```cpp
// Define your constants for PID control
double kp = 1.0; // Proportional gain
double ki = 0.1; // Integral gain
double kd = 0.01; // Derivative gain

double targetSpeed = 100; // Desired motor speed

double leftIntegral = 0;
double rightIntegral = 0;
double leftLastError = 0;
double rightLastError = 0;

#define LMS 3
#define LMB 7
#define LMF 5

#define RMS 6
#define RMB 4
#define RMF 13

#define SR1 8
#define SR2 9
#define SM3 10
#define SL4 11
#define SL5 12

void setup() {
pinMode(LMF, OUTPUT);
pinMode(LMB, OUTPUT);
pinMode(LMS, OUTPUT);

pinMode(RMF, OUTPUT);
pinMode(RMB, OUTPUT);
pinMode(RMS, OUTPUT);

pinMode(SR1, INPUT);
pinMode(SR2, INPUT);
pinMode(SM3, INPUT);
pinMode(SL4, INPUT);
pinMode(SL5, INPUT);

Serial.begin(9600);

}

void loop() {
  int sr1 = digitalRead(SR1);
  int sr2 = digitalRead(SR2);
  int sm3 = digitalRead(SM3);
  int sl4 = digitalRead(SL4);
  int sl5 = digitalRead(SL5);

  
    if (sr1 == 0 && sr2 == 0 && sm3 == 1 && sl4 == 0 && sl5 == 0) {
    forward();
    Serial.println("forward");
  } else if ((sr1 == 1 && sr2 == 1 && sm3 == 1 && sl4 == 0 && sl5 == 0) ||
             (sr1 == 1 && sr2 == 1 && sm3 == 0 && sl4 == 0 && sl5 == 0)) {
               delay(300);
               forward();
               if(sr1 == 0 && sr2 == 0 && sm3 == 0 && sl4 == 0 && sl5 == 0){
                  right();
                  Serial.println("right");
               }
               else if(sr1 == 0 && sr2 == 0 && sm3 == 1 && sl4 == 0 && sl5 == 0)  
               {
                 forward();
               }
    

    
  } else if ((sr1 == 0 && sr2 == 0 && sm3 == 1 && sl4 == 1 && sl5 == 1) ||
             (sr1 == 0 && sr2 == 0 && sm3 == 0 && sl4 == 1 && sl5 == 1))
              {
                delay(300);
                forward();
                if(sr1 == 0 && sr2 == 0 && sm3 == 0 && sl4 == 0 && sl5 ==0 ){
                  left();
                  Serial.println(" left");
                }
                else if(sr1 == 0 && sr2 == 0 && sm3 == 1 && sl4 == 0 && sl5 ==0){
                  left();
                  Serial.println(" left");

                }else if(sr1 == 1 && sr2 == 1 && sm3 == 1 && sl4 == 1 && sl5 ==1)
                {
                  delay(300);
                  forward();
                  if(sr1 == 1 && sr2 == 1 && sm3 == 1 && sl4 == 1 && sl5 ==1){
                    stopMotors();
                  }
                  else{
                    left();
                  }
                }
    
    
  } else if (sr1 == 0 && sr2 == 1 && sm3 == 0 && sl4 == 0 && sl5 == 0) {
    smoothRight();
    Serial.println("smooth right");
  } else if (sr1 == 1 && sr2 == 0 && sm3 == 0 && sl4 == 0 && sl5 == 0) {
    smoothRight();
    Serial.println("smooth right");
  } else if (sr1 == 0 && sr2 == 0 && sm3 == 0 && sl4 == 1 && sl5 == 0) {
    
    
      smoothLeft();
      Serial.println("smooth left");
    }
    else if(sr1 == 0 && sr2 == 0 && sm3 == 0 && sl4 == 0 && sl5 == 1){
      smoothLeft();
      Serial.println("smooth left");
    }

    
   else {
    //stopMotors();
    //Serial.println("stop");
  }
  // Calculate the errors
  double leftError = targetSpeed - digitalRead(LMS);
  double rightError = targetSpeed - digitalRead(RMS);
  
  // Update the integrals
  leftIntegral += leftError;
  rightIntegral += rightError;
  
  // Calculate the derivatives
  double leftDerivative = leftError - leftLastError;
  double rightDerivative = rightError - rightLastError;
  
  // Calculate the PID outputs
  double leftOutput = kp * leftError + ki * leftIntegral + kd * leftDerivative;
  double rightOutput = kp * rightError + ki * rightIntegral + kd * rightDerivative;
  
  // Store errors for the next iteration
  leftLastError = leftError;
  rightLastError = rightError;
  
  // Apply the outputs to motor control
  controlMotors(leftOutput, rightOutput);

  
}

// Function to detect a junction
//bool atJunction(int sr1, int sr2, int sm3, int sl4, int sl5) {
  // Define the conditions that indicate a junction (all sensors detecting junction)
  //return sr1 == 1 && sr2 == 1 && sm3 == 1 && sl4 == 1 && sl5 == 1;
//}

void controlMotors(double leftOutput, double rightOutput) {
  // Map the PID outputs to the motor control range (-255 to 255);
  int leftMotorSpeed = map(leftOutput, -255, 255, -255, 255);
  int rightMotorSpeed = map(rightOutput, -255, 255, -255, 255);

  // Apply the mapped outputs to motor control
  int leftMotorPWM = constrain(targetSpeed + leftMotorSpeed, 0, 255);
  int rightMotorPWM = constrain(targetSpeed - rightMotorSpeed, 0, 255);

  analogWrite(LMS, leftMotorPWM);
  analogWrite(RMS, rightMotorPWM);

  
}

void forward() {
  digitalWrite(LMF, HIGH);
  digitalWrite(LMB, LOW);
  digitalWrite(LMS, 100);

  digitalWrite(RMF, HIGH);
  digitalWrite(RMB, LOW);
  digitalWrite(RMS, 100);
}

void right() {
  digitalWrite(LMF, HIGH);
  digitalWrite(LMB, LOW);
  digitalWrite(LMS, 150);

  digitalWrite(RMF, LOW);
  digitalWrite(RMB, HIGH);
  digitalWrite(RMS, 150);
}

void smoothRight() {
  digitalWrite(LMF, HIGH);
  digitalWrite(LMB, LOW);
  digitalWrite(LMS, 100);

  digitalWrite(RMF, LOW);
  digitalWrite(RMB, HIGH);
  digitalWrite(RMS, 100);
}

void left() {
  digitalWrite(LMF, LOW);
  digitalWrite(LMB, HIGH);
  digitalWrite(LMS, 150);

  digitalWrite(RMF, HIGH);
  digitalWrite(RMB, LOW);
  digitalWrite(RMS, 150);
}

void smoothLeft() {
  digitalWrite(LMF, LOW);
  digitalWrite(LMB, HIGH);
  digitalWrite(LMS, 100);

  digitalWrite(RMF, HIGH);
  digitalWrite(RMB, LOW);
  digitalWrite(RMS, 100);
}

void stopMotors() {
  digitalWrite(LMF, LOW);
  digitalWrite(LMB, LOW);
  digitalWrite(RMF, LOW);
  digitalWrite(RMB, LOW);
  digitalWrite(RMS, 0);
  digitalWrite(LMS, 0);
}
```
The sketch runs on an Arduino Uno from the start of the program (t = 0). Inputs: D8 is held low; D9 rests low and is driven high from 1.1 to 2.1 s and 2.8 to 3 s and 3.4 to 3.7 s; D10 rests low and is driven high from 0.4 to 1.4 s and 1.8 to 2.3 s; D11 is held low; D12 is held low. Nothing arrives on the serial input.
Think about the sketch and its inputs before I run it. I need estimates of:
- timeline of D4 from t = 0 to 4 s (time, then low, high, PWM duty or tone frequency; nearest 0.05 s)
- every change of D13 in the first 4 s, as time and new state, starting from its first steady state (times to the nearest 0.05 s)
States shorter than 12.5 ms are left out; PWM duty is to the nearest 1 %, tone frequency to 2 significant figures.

0 s low; 1.4 s high; 2.1 s low; 2.8 s high
0 s low; 0.4 s high; 1.4 s low; 2.1 s high; 2.8 s low
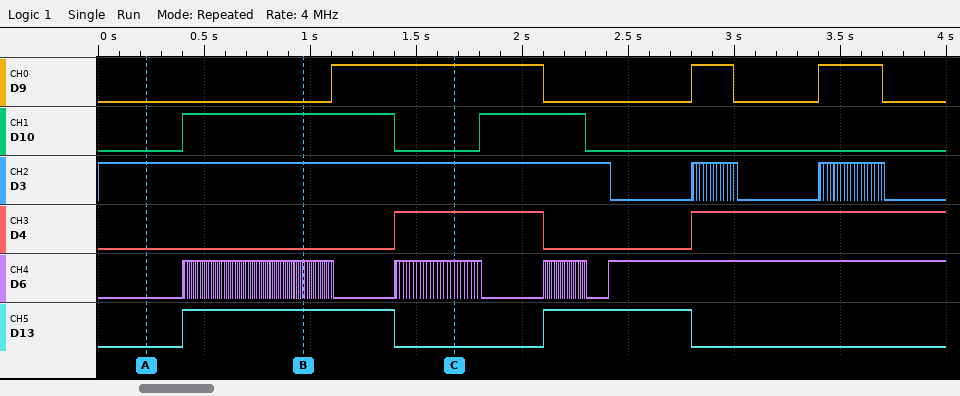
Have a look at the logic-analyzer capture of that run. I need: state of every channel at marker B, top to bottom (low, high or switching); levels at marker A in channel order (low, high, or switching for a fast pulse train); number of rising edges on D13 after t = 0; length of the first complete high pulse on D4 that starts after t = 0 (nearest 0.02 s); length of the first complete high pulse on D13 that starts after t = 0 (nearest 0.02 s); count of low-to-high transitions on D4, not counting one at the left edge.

D9 low, D10 high, D3 high, D4 low, D6 switching, D13 high
D9 low, D10 low, D3 high, D4 low, D6 low, D13 low
2
0.70 s
1.00 s
2
